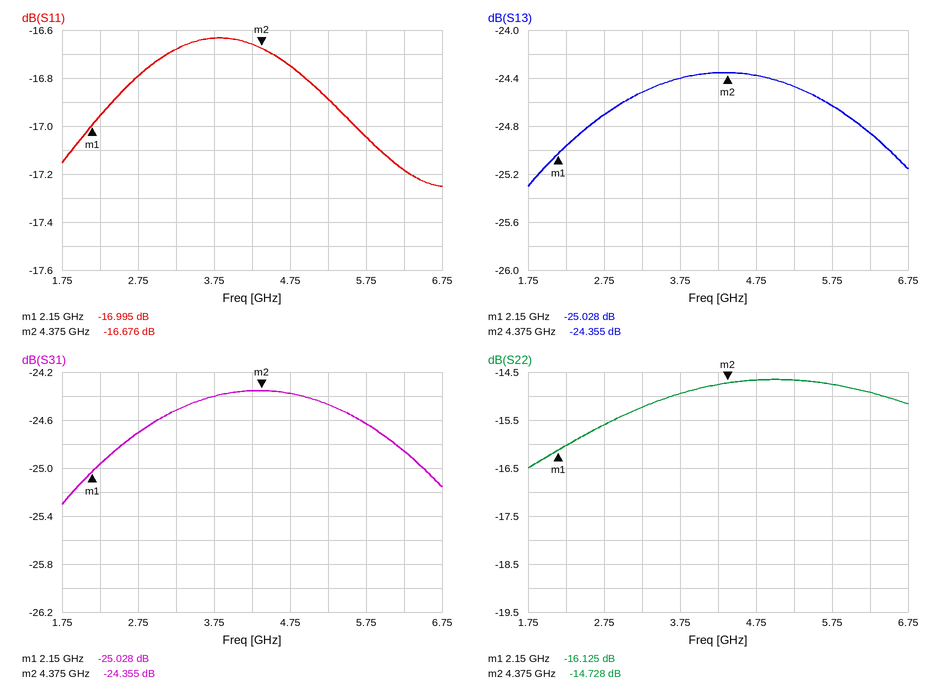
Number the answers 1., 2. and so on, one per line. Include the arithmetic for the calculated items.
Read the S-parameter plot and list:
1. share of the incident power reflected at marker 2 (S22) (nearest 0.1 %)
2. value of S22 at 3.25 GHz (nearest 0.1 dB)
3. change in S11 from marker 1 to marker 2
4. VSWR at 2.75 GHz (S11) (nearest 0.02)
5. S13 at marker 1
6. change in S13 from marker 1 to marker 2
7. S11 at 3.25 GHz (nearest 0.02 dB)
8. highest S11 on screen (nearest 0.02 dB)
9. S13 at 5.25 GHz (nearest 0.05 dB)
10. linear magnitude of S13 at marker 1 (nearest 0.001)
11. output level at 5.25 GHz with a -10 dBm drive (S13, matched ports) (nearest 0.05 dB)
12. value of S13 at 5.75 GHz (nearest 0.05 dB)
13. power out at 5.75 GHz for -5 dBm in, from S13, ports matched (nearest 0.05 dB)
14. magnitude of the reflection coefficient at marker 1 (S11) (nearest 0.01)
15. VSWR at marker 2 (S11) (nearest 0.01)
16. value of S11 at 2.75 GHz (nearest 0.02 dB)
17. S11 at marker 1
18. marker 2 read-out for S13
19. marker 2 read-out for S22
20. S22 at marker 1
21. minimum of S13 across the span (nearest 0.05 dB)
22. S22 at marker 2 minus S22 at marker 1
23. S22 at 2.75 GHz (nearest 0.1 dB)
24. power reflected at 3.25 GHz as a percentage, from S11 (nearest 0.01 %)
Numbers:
1. 10^(-14.728/10) ≈ 3.4 %
2. -15.2 dB
3. -16.676 − (-16.995) = 0.319 dB
4. |Γ| = 10^(-16.8/20) = 0.1445; VSWR = (1 + 0.1445)/(1 − 0.1445) ≈ 1.34
5. -25.028 dB
6. -24.355 − (-25.028) = 0.673 dB
7. -16.68 dB
8. -16.64 dB
9. -24.45 dB
10. 10^(-25.028/20) ≈ 0.056
11. -10 dBm + (-24.45 dB) = -34.45 dBm
12. -24.65 dB
13. -5 dBm + (-24.65 dB) = -29.65 dBm
14. 10^(-16.995/20) ≈ 0.14
15. (1 + 0.1466)/(1 − 0.1466) ≈ 1.34
16. -16.80 dB
17. -16.995 dB
18. -24.355 dB
19. -14.728 dB
20. -16.125 dB
21. -25.30 dB
22. -14.728 − (-16.125) = 1.397 dB
23. -15.6 dB
24. 10^(-16.68/10) ≈ 2.15 %
